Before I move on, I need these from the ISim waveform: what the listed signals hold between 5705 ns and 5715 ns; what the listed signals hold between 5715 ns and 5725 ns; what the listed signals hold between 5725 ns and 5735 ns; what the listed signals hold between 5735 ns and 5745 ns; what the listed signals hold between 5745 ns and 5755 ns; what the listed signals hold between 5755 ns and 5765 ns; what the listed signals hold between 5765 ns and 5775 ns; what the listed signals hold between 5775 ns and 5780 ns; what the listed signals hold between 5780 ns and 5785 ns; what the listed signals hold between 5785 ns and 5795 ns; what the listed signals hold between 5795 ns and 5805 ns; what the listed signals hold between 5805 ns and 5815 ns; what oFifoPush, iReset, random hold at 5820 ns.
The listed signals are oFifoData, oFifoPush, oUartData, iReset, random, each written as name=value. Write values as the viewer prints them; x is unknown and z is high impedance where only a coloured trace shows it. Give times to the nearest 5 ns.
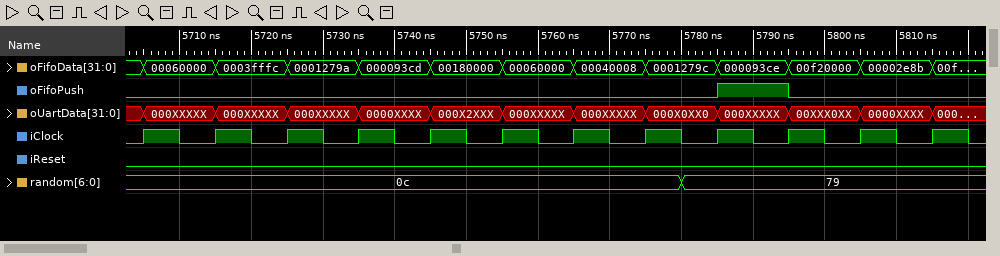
oFifoData=00060000, oFifoPush=0, oUartData=000XXXXX, iReset=0, random=0c
oFifoData=0003fffc, oFifoPush=0, oUartData=000XXXXX, iReset=0, random=0c
oFifoData=0001279a, oFifoPush=0, oUartData=000XXXXX, iReset=0, random=0c
oFifoData=000093cd, oFifoPush=0, oUartData=0000XXXX, iReset=0, random=0c
oFifoData=00180000, oFifoPush=0, oUartData=000X2XXX, iReset=0, random=0c
oFifoData=00060000, oFifoPush=0, oUartData=000XXXXX, iReset=0, random=0c
oFifoData=00040008, oFifoPush=0, oUartData=000XXXXX, iReset=0, random=0c
oFifoData=0001279c, oFifoPush=0, oUartData=000X0XX0, iReset=0, random=0c
oFifoData=0001279c, oFifoPush=0, oUartData=000X0XX0, iReset=0, random=79
oFifoData=000093ce, oFifoPush=1, oUartData=000XXXXX, iReset=0, random=79
oFifoData=00f20000, oFifoPush=0, oUartData=00XXX0XX, iReset=0, random=79
oFifoData=00002e8b, oFifoPush=0, oUartData=0000XXXX, iReset=0, random=79
oFifoPush=0, iReset=0, random=79
